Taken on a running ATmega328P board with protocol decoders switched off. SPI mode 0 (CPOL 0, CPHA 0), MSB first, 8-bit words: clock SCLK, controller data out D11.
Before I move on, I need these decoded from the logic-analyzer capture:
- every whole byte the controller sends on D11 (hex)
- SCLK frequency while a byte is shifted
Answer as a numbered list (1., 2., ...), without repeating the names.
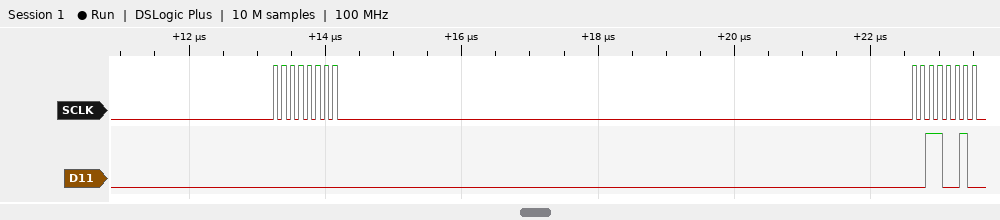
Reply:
1. 0x00 0x32
2. 8 MHz
